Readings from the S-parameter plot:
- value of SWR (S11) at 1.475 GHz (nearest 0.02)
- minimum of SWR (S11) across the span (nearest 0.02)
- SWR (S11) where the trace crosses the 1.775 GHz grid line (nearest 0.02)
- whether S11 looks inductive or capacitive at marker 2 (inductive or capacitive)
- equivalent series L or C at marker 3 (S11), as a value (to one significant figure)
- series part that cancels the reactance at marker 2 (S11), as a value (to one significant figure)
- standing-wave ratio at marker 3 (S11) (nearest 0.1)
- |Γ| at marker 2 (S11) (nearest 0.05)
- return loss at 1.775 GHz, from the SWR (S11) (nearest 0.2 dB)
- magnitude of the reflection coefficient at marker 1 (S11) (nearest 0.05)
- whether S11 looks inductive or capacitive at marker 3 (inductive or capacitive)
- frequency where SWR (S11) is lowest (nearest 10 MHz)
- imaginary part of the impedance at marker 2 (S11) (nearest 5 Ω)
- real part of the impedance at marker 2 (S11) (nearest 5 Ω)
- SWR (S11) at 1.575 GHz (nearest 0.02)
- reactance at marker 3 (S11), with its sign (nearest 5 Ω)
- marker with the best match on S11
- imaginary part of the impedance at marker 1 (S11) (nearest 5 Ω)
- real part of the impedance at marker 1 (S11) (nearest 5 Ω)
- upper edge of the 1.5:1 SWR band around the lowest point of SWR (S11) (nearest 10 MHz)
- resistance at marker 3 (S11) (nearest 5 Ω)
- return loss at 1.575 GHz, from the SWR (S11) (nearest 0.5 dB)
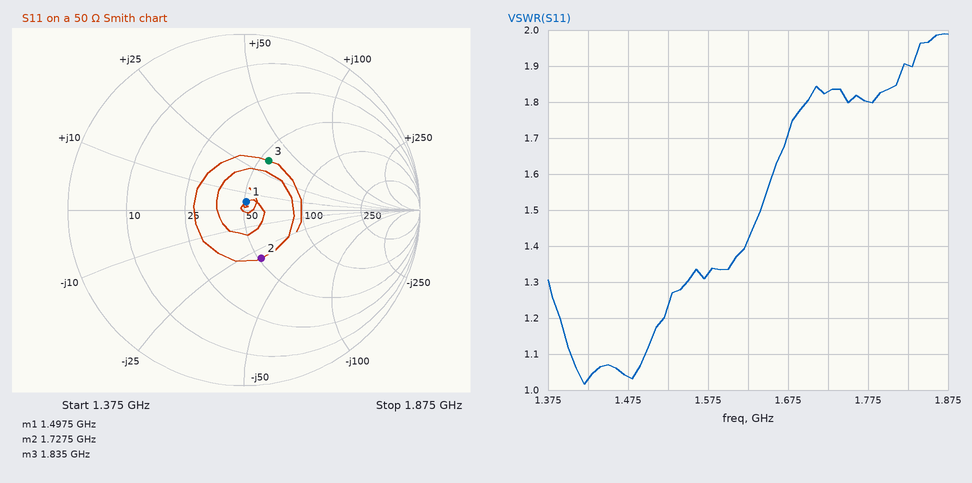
1.04
1.02
1.80
capacitive
3 nH
3 nH
1.9
0.30
10.8 dB
0.05
inductive
1.42 GHz
-30 Ω
50 Ω
1.32
+35 Ω
marker 1
+5 Ω
50 Ω
1.64 GHz
55 Ω
17.0 dB
